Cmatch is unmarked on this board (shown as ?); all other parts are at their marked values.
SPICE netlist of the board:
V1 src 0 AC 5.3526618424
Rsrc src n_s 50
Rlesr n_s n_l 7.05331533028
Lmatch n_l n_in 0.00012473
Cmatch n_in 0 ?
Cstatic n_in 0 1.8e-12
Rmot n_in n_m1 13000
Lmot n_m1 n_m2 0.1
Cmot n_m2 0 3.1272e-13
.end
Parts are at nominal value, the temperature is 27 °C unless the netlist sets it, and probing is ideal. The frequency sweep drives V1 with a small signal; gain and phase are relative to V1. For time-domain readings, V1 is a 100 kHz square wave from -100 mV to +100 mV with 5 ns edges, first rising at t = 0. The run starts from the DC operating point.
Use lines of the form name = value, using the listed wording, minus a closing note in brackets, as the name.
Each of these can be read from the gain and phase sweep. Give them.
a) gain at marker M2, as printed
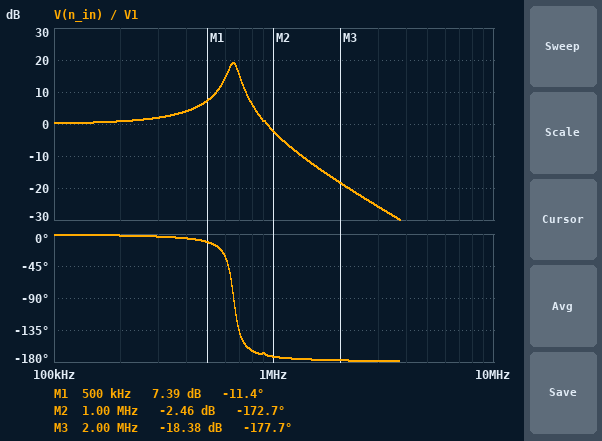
gain at marker M2, as printed = -2.46 dB
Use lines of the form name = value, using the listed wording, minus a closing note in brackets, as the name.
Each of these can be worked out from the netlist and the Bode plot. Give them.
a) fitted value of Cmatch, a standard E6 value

fitted value of Cmatch, a standard E6 value = 470 pF
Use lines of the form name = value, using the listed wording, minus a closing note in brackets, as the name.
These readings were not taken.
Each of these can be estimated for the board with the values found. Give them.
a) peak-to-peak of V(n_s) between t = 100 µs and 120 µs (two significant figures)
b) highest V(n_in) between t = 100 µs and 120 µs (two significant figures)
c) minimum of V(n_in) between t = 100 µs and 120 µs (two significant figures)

peak-to-peak of V(n_s) between t = 100 µs and 120 µs = 230 mV
highest V(n_in) between t = 100 µs and 120 µs = 260 mV
minimum of V(n_in) between t = 100 µs and 120 µs = -260 mV
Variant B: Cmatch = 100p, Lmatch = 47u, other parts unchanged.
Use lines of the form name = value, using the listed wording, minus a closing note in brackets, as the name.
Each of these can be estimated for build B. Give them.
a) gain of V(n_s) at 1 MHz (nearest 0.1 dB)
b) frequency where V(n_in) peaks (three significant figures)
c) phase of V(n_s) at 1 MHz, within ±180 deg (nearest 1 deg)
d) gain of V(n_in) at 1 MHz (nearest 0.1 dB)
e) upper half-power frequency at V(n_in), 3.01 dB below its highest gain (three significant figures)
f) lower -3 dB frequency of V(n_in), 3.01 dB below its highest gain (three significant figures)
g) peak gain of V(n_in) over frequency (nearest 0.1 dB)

gain of V(n_s) at 1 MHz = 0 dB
frequency where V(n_in) peaks = 2.30 MHz
phase of V(n_s) at 1 MHz, within ±180 deg = -2 deg
gain of V(n_in) at 1 MHz = 1.8 dB
upper half-power frequency at V(n_in), 3.01 dB below its highest gain = 2.39 MHz
lower -3 dB frequency of V(n_in), 3.01 dB below its highest gain = 2.20 MHz
peak gain of V(n_in) over frequency = 21.5 dB
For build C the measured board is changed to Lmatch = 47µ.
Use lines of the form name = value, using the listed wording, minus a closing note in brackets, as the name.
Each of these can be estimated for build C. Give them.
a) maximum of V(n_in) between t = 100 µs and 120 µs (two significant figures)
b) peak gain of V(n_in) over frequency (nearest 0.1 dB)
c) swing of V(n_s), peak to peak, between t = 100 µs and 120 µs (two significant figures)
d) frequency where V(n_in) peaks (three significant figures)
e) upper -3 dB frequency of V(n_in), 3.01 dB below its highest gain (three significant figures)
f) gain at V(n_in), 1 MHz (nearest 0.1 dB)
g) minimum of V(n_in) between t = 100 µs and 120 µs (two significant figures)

maximum of V(n_in) between t = 100 µs and 120 µs = 250 mV
peak gain of V(n_in) over frequency = 14.9 dB
swing of V(n_s), peak to peak, between t = 100 µs and 120 µs = 240 mV
frequency where V(n_in) peaks = 1.06 MHz
upper -3 dB frequency of V(n_in), 3.01 dB below its highest gain = 1.15 MHz
gain at V(n_in), 1 MHz = 13.5 dB
minimum of V(n_in) between t = 100 µs and 120 µs = -250 mV
